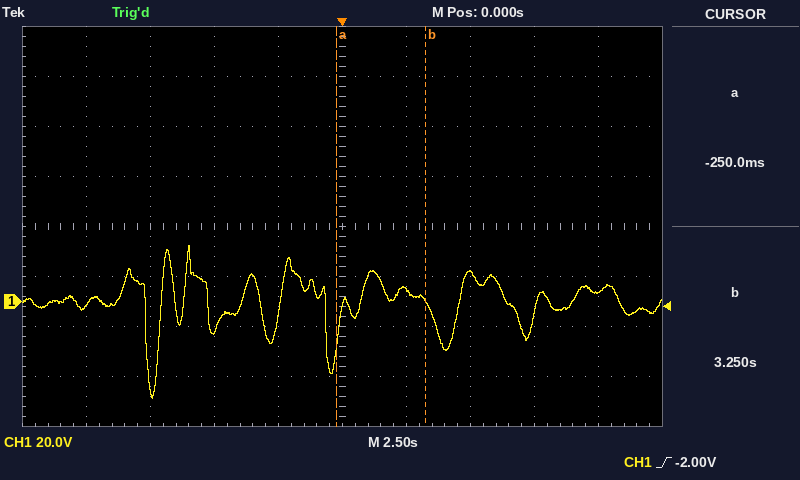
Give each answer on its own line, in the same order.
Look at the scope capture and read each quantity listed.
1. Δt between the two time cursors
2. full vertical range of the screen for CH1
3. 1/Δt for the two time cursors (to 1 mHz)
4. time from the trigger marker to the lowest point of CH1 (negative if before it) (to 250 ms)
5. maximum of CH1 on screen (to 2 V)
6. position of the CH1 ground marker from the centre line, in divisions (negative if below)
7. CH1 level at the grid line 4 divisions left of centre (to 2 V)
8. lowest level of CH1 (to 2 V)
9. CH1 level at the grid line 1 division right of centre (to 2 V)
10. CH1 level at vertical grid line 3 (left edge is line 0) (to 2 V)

3.50 s
160 V
286 mHz
-7.50 s
22 V
-1.5 div
-2 V
-38 V
4 V
-12 V
